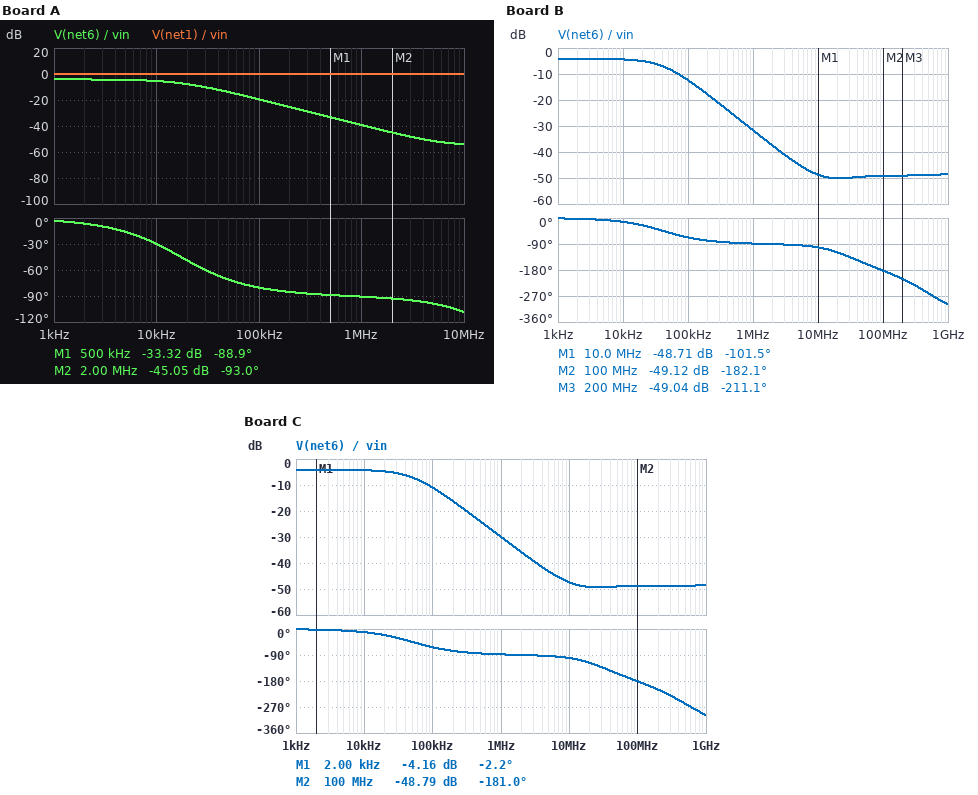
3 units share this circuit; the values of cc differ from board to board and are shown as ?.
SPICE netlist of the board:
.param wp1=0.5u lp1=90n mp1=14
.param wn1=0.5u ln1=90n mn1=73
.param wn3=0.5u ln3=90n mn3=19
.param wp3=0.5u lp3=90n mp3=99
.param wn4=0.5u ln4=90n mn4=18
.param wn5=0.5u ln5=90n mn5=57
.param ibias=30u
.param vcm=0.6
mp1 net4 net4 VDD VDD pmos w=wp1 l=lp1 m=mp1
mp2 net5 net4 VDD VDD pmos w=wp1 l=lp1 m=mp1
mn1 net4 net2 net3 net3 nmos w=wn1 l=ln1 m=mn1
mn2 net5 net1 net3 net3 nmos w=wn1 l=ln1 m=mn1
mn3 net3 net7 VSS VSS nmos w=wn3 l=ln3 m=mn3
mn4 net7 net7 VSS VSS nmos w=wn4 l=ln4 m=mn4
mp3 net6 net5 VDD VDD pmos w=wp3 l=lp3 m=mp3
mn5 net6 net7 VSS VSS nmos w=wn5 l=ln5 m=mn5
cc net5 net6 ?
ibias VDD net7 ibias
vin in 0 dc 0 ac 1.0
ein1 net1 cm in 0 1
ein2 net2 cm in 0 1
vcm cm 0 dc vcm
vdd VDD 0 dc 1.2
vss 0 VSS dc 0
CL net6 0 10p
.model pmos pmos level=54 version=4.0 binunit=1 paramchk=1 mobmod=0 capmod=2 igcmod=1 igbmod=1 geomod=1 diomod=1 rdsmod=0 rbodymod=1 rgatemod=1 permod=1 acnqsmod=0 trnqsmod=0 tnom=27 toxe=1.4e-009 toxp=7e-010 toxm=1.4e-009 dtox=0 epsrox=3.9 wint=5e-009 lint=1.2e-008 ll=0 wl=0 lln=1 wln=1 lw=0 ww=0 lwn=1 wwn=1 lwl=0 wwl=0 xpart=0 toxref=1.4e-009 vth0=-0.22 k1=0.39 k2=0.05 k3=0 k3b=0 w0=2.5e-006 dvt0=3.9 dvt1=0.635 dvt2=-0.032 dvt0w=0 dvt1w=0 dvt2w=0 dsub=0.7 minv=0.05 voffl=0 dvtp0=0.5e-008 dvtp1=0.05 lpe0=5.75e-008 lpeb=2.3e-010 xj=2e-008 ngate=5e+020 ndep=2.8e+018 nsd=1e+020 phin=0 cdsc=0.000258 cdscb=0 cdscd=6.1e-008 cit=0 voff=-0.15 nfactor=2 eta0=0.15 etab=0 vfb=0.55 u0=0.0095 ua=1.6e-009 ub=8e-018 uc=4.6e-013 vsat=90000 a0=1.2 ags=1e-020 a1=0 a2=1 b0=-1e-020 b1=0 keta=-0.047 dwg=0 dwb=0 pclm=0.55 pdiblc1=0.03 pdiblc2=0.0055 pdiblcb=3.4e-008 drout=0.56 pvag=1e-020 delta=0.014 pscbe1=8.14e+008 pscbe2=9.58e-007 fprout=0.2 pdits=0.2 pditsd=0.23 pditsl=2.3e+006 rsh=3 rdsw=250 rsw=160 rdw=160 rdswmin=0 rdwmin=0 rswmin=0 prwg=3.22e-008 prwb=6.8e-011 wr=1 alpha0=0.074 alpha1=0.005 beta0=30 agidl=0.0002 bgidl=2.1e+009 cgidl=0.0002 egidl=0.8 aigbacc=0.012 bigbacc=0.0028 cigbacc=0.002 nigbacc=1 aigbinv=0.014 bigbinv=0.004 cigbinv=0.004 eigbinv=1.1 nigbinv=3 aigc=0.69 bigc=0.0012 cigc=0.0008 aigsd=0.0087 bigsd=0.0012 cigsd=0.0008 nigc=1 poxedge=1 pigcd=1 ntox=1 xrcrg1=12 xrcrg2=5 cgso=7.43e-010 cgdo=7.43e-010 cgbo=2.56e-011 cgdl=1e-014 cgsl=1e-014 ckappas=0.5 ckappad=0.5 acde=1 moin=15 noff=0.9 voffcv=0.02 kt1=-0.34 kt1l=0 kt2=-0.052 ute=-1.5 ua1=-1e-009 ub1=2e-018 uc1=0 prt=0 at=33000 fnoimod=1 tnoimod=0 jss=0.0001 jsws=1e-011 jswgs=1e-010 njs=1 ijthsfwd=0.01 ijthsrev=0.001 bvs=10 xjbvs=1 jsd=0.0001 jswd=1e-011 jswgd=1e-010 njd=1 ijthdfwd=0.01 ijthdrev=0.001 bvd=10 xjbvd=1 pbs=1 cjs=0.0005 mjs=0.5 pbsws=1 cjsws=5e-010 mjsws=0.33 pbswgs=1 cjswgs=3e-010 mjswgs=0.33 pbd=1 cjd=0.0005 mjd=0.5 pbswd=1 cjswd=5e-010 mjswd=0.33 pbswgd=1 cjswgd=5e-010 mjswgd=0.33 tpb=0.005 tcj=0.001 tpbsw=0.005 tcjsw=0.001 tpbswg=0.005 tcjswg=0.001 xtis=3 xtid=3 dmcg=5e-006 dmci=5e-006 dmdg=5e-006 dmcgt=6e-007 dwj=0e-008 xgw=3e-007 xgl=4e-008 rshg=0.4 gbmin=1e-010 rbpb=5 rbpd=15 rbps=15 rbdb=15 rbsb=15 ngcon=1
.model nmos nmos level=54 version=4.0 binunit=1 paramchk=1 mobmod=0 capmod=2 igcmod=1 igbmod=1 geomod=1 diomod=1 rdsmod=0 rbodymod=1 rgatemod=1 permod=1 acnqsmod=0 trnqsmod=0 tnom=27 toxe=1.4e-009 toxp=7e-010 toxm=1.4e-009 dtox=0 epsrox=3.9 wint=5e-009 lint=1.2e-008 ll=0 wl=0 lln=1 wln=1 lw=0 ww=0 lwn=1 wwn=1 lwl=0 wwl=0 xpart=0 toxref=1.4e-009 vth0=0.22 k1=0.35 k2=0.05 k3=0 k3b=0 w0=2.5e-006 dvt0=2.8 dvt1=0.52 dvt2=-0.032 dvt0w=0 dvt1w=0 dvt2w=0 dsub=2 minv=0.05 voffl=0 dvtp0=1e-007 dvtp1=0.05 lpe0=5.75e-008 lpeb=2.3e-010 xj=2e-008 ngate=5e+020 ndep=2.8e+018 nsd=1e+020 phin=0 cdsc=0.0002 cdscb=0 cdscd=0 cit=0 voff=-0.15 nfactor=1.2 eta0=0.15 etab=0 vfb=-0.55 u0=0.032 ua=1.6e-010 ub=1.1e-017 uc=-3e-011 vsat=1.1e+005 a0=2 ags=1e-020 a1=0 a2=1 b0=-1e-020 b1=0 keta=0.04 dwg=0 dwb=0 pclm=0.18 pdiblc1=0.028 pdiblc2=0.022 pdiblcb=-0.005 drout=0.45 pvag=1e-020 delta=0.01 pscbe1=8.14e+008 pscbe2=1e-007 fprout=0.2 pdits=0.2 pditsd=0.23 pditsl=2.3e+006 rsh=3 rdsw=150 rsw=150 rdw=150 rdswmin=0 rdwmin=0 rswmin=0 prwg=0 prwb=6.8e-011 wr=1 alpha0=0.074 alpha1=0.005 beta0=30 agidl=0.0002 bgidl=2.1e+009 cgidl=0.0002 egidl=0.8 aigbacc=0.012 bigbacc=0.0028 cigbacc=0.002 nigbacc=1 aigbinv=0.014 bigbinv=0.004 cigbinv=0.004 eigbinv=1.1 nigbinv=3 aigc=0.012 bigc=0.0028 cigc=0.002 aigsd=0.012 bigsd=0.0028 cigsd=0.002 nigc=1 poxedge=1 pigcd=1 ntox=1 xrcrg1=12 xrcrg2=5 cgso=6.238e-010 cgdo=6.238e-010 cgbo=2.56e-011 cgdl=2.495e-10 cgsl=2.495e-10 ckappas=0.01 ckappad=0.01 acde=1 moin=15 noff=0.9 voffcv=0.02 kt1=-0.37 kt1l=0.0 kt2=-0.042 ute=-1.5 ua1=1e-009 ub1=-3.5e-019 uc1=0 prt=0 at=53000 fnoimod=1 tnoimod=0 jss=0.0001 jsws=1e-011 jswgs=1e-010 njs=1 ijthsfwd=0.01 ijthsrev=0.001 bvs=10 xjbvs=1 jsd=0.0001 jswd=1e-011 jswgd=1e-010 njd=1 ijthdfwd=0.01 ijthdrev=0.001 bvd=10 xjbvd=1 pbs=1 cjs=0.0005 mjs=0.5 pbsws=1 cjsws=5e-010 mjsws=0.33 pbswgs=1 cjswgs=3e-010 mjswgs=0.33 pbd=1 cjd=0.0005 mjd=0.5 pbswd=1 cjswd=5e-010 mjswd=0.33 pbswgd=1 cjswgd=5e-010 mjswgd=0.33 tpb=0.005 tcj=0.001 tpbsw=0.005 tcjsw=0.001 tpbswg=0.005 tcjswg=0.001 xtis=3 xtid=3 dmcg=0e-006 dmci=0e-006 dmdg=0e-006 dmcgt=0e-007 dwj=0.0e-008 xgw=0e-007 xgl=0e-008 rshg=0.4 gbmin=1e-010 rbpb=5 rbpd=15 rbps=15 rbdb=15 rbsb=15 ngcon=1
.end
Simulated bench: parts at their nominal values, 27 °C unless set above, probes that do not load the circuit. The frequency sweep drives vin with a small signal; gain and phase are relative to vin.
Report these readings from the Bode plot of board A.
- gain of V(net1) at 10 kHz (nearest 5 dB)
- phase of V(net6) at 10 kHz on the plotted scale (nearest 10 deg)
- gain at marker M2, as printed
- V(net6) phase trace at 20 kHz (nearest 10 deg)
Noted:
0 dB
-30 deg
-45.05 dB
-50 deg
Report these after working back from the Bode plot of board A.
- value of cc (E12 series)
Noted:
8.2 pF
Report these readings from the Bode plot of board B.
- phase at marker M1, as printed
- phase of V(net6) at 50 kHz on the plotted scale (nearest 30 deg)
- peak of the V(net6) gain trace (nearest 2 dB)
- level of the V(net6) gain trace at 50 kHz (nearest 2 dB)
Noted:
-101.5 deg
-60 deg
-4 dB
-8 dB
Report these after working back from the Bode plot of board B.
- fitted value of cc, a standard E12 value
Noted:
3.3 pF
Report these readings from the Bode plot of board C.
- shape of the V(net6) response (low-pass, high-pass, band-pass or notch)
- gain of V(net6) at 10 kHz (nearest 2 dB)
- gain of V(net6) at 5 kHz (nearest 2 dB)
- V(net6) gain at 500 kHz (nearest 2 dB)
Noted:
low-pass
-4 dB
-4 dB
-24 dB
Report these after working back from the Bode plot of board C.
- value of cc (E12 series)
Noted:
2.7 pF
